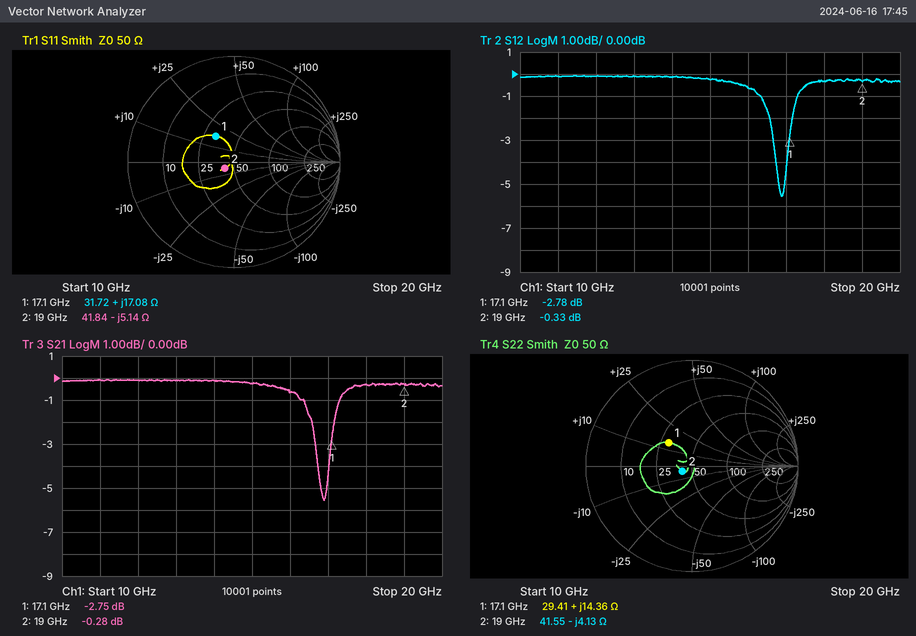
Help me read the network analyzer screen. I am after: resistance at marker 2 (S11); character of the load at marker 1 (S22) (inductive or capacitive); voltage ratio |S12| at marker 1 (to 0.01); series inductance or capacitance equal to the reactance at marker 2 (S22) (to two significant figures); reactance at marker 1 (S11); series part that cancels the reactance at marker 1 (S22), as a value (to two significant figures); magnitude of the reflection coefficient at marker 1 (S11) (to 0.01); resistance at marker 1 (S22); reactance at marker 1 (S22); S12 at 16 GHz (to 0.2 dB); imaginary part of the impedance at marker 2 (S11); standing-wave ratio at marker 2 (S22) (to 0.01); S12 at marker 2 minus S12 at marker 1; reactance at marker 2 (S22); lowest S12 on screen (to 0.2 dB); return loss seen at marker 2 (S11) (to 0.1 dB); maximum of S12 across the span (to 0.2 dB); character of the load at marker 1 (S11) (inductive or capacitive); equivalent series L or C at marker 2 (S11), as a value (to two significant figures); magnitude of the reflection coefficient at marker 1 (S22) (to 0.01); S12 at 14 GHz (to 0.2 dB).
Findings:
41.84 Ω
inductive
0.73
2.0 pF
+17.08 Ω
650 fF
0.30
29.41 Ω
+14.36 Ω
-0.6 dB
-5.14 Ω
1.23
2.45 dB
-4.13 Ω
-5.6 dB
19.6 dB
0.0 dB
inductive
1.6 pF
0.31
-0.2 dB
